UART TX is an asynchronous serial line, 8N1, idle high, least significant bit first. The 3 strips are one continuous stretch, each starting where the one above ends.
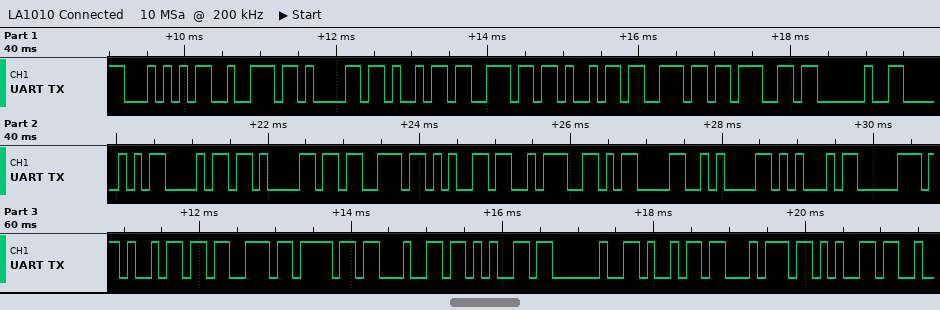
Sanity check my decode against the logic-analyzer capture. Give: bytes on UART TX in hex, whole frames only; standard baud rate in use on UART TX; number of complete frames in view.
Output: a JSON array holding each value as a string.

["54 72 61 69 6E 69 6E 67 20 50 68 61 73 65 3A 0D 0A 45 70 69 73 6F 64 65 20 69 74 65", "9600 baud", "28"]
